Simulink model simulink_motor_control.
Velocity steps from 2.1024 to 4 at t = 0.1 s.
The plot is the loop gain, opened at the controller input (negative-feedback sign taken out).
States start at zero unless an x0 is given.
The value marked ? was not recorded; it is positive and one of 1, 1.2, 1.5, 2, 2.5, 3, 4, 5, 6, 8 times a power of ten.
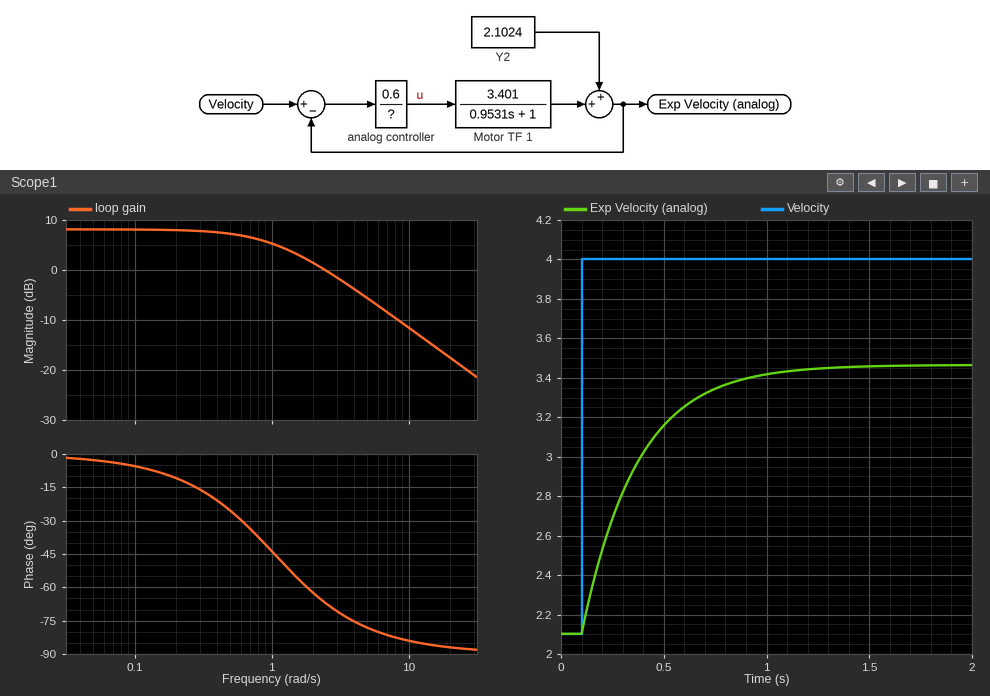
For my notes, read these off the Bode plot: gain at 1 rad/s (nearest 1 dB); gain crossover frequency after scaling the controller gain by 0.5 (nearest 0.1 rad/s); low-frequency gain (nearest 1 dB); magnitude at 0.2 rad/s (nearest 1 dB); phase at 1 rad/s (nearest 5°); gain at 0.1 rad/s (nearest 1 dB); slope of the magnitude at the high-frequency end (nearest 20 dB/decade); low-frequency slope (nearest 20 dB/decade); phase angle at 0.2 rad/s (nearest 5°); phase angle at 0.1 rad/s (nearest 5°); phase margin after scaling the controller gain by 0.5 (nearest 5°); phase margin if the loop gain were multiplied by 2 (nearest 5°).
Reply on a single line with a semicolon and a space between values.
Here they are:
5 dB; 0.8 rad/s; 8 dB; 8 dB; -45°; 8 dB; -20 dB/decade; 0 dB/decade; -10°; -5°; 140°; 100°
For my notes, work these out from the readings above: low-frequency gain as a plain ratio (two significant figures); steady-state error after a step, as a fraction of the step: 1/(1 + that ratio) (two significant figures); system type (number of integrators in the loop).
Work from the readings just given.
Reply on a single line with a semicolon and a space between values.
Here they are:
2.5; 0.29; 0
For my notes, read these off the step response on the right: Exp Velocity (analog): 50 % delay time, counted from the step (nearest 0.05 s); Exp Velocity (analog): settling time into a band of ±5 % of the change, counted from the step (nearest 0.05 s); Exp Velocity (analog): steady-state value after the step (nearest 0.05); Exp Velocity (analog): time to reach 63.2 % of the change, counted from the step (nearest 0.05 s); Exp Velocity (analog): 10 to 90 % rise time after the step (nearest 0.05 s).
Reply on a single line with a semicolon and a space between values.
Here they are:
0.20 s; 0.80 s; 3.45; 0.25 s; 0.60 s
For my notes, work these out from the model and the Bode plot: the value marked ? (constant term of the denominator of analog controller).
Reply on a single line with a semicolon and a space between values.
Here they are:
0.8
